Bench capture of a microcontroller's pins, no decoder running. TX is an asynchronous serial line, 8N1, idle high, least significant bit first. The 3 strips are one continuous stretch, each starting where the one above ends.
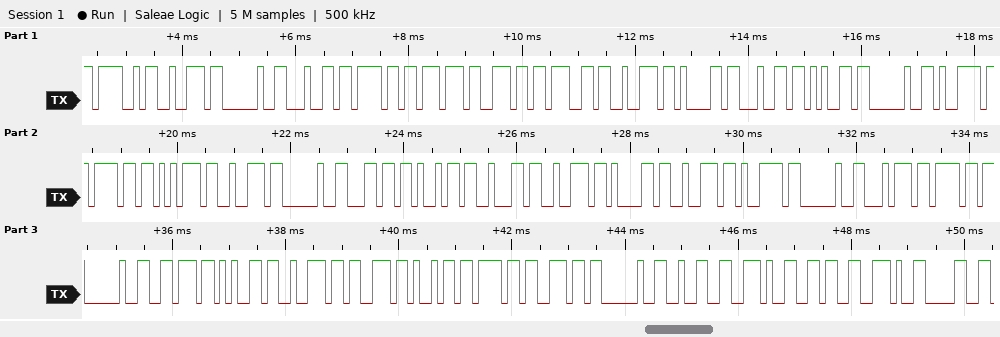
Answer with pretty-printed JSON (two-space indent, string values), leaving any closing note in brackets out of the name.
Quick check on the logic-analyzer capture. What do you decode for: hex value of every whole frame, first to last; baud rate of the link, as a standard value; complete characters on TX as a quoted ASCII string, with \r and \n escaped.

{
  "hex value of every whole frame, first to last": "0x4F 0x72 0x20 0x64 0x6F 0x77 0x6E 0x67 0x72 0x61 0x64 0x65 0x20 0x79 0x6F 0x75 0x72 0x20 0x6C 0x69 0x62 0x72 0x61 0x72 0x79 0x20 0x74 0x6F 0x20 0x76 0x65 0x72 0x73 0x69 0x6F 0x6E 0x20 0x32 0x2E 0x36 0x2E 0x30",
  "baud rate of the link, as a standard value": "9600 baud",
  "complete characters on TX as a quoted ASCII string, with \\r and \\n escaped": "\"Or downgrade your library to version 2.6.0\""
}
